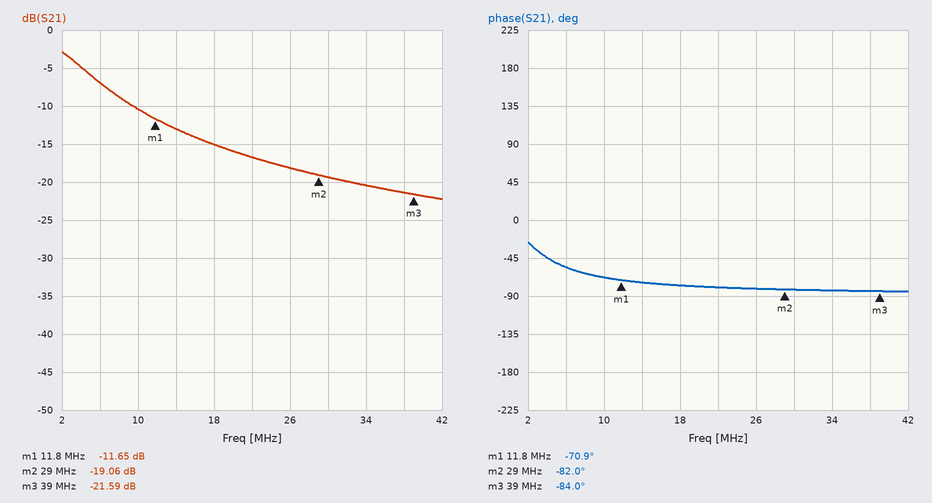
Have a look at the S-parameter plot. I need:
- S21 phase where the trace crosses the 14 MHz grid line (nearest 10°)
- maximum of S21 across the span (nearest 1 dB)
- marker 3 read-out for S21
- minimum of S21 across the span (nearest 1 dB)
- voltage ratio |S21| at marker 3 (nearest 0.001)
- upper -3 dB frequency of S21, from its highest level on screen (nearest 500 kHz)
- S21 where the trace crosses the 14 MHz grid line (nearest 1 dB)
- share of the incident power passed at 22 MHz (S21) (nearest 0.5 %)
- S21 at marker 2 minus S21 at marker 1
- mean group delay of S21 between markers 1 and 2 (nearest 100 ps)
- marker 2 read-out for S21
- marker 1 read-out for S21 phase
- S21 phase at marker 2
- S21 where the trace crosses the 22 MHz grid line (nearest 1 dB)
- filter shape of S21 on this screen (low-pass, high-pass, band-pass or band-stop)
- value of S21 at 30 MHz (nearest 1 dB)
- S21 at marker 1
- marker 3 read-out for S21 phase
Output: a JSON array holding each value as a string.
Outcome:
["-70°", "-3 dB", "-21.59 dB", "-22 dB", "0.083", "5.0 MHz", "-13 dB", "2.0 %", "-7.41 dB", "1.8 ns", "-19.06 dB", "-70.9°", "-82.0°", "-17 dB", "low-pass", "-19 dB", "-11.65 dB", "-84.0°"]
